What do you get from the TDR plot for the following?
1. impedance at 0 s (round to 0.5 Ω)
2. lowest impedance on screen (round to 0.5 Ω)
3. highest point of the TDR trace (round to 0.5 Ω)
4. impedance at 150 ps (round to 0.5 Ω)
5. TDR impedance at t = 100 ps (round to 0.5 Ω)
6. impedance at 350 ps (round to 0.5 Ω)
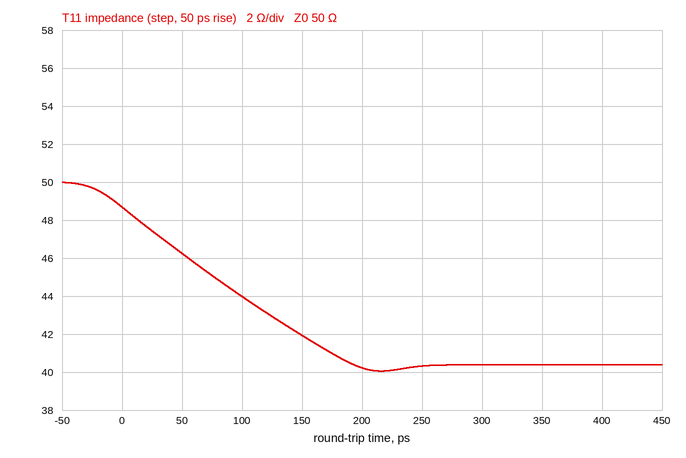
48.5 Ω
40.0 Ω
50.0 Ω
42.0 Ω
44.0 Ω
40.5 Ω
